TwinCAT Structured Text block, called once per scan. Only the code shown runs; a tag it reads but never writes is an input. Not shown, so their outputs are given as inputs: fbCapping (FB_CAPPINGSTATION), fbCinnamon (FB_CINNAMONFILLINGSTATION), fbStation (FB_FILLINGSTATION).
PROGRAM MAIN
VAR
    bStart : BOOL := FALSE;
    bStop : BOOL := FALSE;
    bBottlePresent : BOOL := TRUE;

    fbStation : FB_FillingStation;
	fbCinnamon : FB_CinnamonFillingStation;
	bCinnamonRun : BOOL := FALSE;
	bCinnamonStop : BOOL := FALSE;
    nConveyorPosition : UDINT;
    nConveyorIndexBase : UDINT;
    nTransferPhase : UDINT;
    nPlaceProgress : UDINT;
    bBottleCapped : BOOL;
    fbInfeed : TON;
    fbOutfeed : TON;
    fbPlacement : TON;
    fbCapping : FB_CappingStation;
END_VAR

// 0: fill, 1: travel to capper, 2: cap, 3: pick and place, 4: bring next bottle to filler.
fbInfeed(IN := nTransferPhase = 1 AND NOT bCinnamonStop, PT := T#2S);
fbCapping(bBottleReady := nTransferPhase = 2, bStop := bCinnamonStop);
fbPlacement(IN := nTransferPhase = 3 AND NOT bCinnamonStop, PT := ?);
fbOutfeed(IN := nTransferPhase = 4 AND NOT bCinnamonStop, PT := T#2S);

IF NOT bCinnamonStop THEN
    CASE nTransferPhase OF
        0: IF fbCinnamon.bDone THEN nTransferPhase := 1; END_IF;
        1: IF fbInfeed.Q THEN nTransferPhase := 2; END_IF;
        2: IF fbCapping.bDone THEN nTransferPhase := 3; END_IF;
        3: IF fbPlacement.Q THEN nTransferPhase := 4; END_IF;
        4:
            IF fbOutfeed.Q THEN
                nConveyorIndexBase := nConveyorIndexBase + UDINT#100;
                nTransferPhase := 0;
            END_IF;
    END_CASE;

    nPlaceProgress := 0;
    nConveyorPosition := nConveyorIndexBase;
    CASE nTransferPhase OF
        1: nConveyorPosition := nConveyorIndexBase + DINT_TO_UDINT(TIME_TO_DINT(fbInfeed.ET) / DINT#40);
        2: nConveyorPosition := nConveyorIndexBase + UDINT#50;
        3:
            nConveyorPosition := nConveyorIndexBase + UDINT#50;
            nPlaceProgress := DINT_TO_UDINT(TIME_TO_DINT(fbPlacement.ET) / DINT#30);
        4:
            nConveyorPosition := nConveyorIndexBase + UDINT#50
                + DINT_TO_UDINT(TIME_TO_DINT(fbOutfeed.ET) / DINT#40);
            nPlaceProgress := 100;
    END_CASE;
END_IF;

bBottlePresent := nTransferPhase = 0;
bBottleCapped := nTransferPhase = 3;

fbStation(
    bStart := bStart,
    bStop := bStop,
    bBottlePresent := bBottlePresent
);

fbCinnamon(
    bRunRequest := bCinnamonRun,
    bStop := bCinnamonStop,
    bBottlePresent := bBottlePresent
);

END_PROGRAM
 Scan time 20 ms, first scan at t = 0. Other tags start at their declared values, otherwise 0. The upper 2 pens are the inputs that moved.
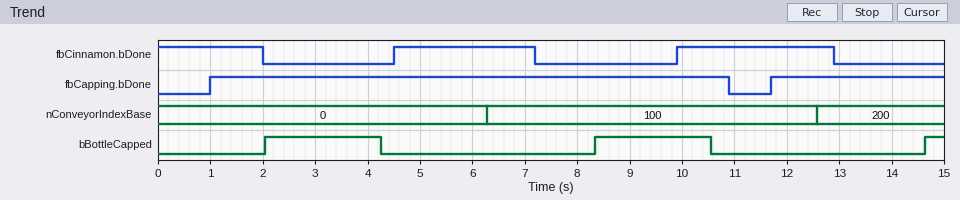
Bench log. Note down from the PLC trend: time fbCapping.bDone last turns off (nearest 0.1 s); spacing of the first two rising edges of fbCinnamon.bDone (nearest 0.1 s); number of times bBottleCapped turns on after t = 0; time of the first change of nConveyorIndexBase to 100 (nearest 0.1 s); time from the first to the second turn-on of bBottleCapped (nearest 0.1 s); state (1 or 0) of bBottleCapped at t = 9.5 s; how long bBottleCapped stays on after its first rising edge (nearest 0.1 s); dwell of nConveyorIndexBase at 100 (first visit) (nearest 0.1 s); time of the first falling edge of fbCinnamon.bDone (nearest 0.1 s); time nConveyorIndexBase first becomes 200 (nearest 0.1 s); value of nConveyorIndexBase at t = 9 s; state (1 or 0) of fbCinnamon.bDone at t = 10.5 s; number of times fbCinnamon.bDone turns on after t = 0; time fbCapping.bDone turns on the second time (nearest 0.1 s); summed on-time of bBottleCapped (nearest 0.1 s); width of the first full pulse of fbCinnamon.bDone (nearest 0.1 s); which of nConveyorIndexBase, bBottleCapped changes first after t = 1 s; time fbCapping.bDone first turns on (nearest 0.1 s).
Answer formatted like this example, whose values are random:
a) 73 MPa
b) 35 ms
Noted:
a) 10.9 s
b) 5.4 s
c) 3
d) 6.3 s
e) 6.3 s
f) 1
g) 2.2 s
h) 6.3 s
i) 2.0 s
j) 12.6 s
k) 100
l) 1
m) 2
n) 11.7 s
o) 4.8 s
p) 2.7 s
q) bBottleCapped
r) 1.0 s
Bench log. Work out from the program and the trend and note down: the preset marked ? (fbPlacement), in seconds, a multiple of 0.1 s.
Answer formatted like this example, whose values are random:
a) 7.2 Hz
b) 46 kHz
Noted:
a) 2.2 s
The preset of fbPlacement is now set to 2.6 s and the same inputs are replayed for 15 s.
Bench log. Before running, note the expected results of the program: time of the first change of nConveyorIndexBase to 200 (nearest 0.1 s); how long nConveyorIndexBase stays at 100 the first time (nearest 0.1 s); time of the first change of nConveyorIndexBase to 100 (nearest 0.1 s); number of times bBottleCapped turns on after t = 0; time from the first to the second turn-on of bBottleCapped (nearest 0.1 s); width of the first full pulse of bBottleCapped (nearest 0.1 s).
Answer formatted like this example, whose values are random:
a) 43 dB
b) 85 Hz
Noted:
a) 13.4 s
b) 6.7 s
c) 6.7 s
d) 2
e) 6.7 s
f) 2.6 s
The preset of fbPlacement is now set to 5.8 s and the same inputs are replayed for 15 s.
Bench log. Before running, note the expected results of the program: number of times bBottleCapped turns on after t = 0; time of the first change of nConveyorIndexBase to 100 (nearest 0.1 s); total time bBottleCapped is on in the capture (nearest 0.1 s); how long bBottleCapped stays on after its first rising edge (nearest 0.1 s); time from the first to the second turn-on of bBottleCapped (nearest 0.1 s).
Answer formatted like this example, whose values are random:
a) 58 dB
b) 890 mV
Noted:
a) 2
b) 9.9 s
c) 8.9 s
d) 5.8 s
e) 9.9 s
